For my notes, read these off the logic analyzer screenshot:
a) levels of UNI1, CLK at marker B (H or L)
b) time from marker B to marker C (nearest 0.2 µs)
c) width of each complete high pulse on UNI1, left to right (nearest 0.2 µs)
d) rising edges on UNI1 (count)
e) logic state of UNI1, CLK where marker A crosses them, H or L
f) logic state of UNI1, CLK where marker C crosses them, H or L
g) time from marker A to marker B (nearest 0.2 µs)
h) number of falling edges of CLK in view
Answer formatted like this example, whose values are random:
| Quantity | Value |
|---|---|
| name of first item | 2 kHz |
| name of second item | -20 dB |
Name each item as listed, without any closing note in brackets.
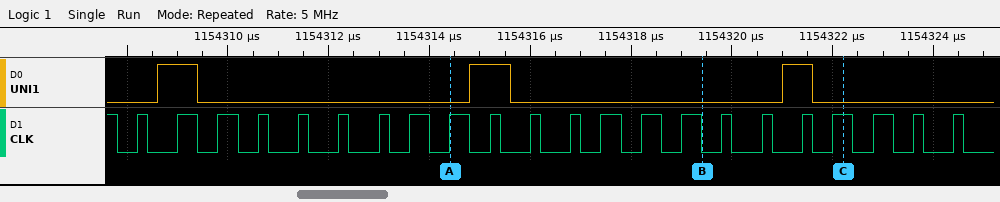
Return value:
| Quantity | Value |
|---|---|
| levels of UNI1, CLK at marker B | UNI1=L, CLK=L |
| time from marker B to marker C | 2.8 µs |
| width of each complete high pulse on UNI1, left to right | 0.8 µs, 0.8 µs, 0.6 µs |
| rising edges on UNI1 | 3 |
| logic state of UNI1, CLK where marker A crosses them, H or L | UNI1=L, CLK=H |
| logic state of UNI1, CLK where marker C crosses them, H or L | UNI1=L, CLK=H |
| time from marker A to marker B | 5 µs |
| number of falling edges of CLK in view | 23 |
